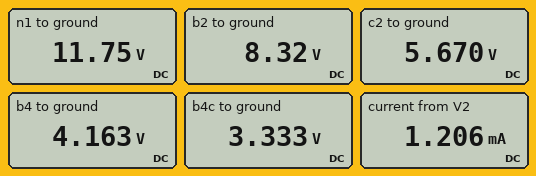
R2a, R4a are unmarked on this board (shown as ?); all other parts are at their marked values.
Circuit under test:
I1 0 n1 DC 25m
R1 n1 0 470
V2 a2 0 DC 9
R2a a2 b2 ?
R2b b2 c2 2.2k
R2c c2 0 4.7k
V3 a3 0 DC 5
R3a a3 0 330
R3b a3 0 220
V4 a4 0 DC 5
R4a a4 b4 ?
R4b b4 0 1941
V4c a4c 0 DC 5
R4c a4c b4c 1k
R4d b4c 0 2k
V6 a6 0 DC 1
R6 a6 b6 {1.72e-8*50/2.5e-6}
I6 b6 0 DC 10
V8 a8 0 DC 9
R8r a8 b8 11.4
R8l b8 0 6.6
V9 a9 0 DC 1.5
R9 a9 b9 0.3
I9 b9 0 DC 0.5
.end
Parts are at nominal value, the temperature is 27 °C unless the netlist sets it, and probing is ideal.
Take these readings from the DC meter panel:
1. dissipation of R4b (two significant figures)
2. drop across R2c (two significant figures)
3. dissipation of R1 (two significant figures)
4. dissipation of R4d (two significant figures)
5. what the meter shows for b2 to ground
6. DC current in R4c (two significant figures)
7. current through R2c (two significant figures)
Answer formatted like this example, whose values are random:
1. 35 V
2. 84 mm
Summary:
1. 8.9 mW
2. 5.7 V
3. 290 mW
4. 5.6 mW
5. 8.32 V
6. 1.7 mA
7. 1.2 mA
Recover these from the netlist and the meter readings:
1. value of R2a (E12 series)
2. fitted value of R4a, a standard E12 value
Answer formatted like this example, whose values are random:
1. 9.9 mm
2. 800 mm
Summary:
1. 560 Ω
2. 390 Ω
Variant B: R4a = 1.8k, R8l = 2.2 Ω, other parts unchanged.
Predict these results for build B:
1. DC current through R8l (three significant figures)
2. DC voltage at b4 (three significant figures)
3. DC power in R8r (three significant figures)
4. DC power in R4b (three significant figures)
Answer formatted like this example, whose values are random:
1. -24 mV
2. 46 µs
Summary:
1. 662 mA
2. 2.59 V
3. 4.99 W
4. 3.47 mW
